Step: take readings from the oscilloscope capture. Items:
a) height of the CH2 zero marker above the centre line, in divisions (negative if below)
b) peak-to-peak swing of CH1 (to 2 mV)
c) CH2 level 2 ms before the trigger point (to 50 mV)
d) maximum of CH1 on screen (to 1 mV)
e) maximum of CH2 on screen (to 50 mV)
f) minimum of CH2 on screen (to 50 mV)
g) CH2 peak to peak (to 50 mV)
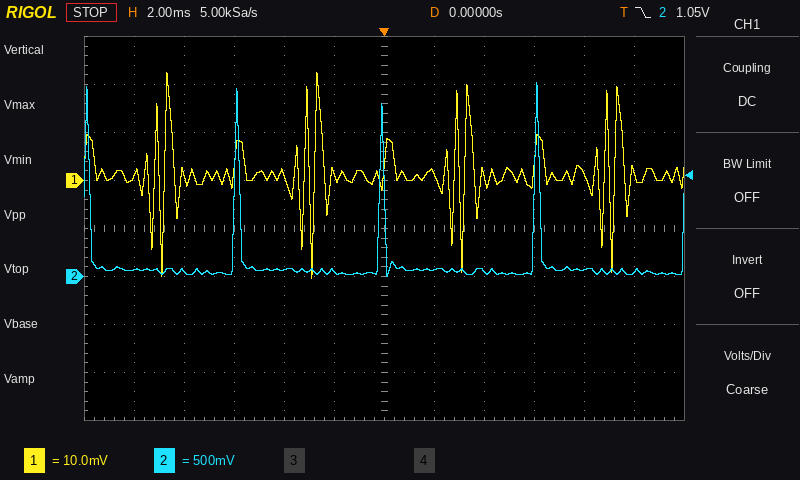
-1.0 div
42 mV
50 mV
22 mV
2.00 V
0 mV
2.00 V
